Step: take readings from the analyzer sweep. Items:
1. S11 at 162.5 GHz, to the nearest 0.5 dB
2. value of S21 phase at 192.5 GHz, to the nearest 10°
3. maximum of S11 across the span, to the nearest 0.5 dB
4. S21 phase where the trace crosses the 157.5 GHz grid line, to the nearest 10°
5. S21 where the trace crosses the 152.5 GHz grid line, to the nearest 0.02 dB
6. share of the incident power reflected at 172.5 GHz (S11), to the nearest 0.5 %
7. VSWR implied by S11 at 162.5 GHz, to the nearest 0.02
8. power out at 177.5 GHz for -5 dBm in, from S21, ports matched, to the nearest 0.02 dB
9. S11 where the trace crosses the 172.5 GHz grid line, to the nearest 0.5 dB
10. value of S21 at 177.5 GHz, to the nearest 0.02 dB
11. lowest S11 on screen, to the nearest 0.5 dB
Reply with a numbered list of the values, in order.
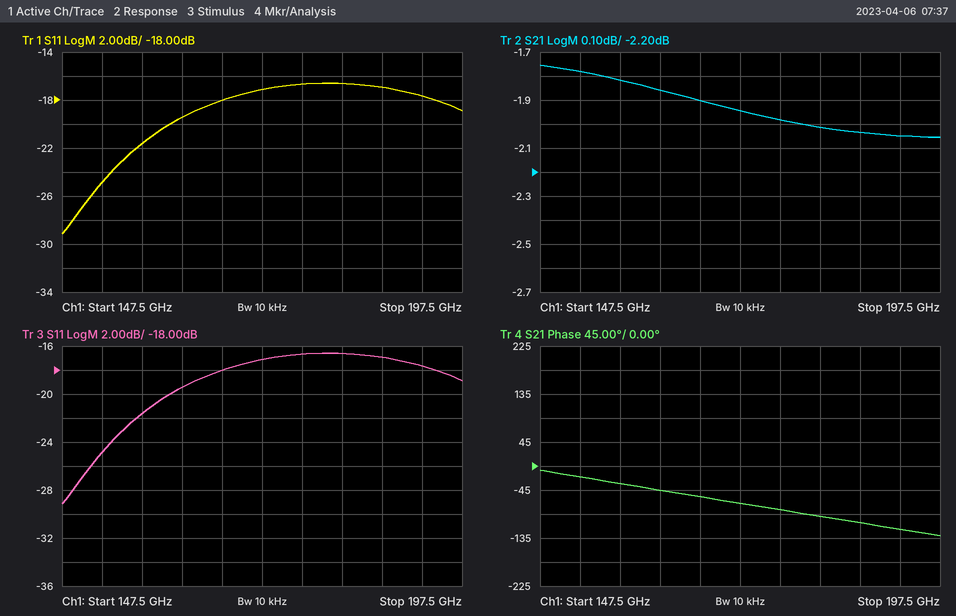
1. -19.5 dB
2. -120°
3. -16.5 dB
4. -30°
5. -1.78 dB
6. 2.0 %
7. 1.24
8. -6.98 dBm
9. -17.0 dB
10. -1.98 dB
11. -29.0 dB
